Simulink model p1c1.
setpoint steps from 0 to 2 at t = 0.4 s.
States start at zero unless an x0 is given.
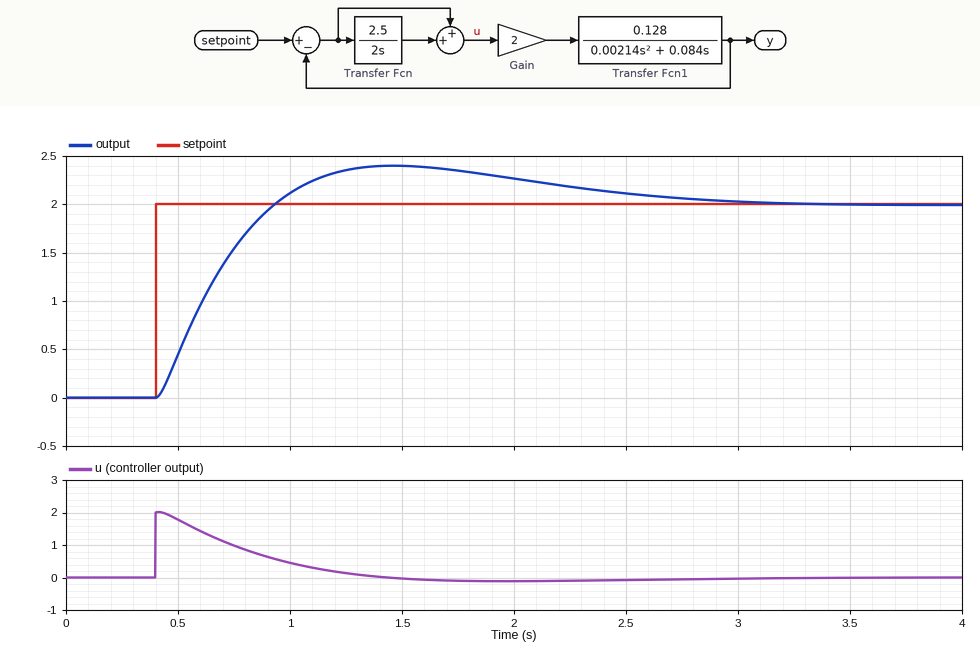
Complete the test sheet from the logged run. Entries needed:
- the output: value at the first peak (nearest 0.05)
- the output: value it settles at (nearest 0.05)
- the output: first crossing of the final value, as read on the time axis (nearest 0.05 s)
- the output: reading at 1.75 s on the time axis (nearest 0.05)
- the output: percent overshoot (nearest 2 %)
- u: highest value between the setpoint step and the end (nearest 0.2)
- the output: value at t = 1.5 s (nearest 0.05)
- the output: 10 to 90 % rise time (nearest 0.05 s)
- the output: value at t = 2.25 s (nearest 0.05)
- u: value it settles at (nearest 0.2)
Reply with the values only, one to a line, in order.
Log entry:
2.40
2.00
0.95 s
2.35
20 %
2.0
2.40
0.40 s
2.20
0.0
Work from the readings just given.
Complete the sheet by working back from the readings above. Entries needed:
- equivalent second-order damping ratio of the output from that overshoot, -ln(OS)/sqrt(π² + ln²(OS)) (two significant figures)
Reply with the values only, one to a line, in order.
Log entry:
0.46
